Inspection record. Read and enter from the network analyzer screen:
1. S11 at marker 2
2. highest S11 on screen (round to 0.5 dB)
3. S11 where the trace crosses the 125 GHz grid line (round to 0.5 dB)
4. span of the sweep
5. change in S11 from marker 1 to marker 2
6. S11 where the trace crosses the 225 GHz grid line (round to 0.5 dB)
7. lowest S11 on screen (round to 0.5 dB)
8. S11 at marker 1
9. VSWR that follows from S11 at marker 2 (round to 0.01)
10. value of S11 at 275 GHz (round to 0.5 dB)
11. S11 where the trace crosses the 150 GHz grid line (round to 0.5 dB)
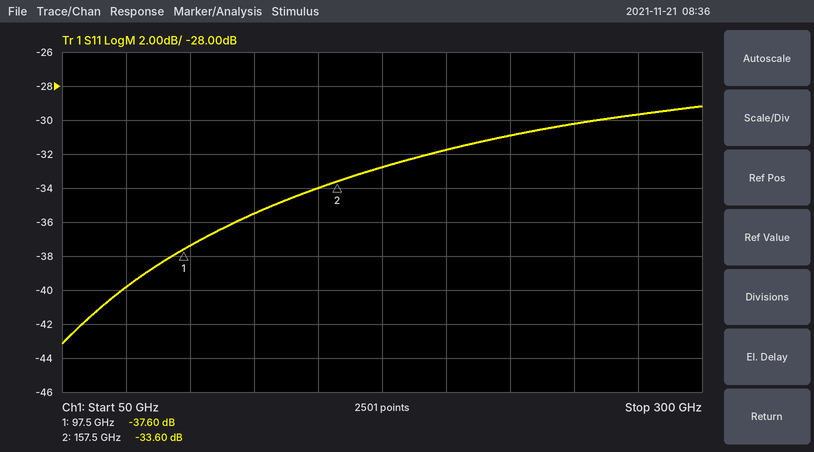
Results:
-33.60 dB
-29.0 dB
-35.5 dB
250 GHz
4.00 dB
-31.0 dB
-43.0 dB
-37.60 dB
1.04
-29.5 dB
-34.0 dB
